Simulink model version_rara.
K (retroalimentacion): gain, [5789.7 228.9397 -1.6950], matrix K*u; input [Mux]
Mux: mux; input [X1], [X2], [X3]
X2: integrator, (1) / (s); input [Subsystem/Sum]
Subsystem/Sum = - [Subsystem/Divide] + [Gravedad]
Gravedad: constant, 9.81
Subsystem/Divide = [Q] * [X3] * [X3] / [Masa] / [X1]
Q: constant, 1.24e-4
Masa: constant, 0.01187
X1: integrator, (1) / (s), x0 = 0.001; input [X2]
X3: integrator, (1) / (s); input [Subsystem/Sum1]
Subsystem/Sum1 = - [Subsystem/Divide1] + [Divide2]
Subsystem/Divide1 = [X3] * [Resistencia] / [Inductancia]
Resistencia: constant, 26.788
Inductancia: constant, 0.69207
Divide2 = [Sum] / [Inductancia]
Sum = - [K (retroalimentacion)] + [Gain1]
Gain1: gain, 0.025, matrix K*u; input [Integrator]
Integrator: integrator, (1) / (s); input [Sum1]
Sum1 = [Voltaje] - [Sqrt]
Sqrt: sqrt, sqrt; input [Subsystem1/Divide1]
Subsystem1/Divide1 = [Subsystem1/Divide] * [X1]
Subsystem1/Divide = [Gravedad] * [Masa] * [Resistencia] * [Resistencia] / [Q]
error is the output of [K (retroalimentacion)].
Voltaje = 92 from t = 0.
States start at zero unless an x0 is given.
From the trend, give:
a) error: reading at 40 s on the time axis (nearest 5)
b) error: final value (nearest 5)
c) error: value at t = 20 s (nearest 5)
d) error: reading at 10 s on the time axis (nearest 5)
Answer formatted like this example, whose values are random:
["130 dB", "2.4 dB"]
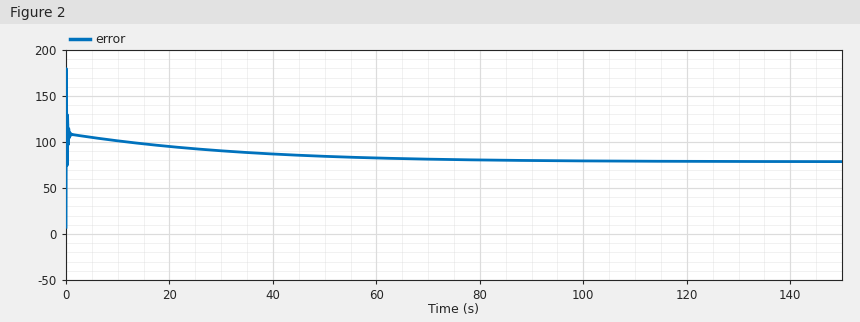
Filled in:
["85", "80", "95", "100"]
